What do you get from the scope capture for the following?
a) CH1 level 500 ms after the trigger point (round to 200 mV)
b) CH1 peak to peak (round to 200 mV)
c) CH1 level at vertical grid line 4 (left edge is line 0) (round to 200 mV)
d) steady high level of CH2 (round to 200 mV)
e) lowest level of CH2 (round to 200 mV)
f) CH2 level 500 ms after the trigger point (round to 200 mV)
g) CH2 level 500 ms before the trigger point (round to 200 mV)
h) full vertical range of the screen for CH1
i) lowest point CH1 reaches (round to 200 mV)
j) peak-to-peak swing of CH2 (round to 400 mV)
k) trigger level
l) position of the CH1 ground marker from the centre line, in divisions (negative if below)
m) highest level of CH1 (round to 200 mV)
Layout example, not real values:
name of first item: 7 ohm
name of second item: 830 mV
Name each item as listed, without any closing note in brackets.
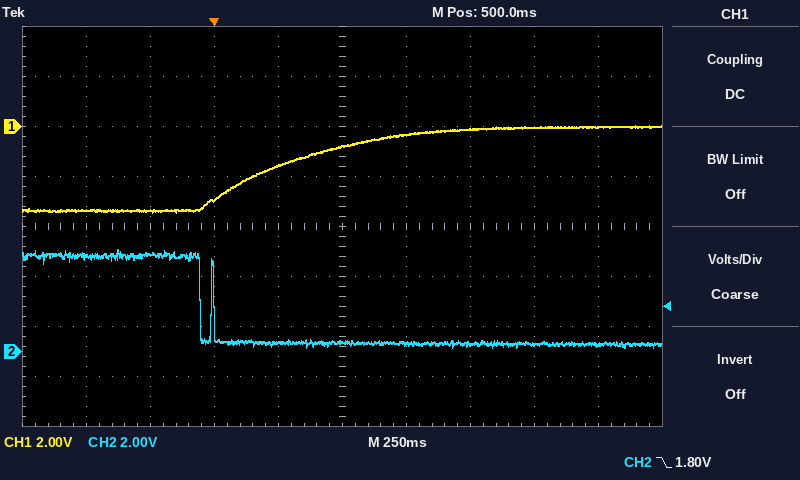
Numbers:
CH1 level 500 ms after the trigger point: -800 mV
CH1 peak to peak: 3.4 V
CH1 level at vertical grid line 4 (left edge is line 0): -1.6 V
steady high level of CH2: 3.8 V
lowest level of CH2: 200 mV
CH2 level 500 ms after the trigger point: 400 mV
CH2 level 500 ms before the trigger point: 3.8 V
full vertical range of the screen for CH1: 16 V
lowest point CH1 reaches: -3.4 V
peak-to-peak swing of CH2: 4.0 V
trigger level: 1.80 V
position of the CH1 ground marker from the centre line, in divisions: +2.0 div
highest level of CH1: 0.0 V
